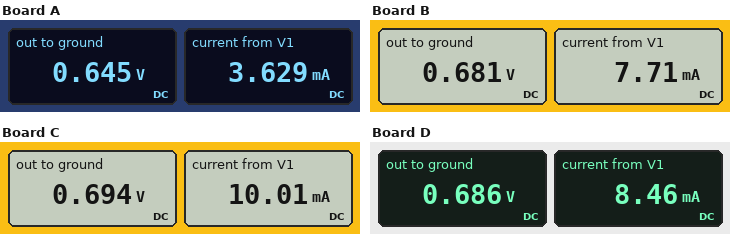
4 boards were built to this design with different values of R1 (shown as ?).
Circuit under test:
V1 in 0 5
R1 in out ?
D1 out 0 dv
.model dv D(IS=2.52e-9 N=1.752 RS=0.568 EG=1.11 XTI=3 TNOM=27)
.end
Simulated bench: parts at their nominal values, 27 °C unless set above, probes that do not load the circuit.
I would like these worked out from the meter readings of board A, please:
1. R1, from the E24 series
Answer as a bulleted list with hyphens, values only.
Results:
- 1.2 kΩ
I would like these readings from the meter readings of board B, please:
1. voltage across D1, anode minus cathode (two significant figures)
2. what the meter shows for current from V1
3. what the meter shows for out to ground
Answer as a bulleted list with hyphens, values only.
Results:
- 680 mV
- 7.71 mA
- 0.681 V
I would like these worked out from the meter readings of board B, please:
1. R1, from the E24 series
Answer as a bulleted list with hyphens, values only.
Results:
- 560 Ω
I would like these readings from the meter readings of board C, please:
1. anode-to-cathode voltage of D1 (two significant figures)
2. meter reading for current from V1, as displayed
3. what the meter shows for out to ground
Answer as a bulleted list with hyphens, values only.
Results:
- 690 mV
- 10.01 mA
- 0.694 V
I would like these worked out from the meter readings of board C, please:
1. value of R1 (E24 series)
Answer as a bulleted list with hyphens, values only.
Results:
- 430 Ω
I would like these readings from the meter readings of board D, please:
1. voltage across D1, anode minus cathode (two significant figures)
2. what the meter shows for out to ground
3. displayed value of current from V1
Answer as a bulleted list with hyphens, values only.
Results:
- 690 mV
- 0.686 V
- 8.46 mA
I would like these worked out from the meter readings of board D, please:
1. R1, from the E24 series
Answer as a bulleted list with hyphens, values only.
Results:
- 510 Ω
